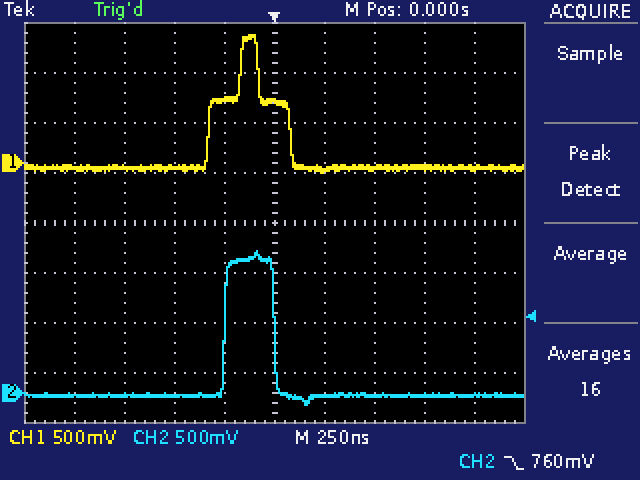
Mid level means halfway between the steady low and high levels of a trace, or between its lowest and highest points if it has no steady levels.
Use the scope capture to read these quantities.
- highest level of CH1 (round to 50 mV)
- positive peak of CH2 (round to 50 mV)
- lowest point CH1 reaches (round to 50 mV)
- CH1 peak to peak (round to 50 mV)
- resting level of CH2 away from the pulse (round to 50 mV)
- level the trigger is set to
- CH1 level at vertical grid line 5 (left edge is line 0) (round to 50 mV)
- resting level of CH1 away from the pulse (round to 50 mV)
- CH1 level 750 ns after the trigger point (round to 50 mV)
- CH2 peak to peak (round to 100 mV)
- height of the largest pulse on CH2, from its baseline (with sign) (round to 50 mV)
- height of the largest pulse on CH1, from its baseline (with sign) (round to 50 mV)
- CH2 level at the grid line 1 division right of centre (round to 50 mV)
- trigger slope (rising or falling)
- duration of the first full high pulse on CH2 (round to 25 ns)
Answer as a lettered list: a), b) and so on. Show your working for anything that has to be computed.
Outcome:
a) 1.30 V
b) 1.40 V
c) -100 mV
d) 1.30 V − (-100 mV) = 1.40 V
e) -50 mV
f) 760 mV
g) 600 mV
h) -50 mV
i) -50 mV
j) 1.50 V
k) 1.40 V − (-50 mV) = +1.45 V
l) 1.30 V − (-50 mV) = +1.35 V
m) -50 mV
n) falling
o) 250 ns
